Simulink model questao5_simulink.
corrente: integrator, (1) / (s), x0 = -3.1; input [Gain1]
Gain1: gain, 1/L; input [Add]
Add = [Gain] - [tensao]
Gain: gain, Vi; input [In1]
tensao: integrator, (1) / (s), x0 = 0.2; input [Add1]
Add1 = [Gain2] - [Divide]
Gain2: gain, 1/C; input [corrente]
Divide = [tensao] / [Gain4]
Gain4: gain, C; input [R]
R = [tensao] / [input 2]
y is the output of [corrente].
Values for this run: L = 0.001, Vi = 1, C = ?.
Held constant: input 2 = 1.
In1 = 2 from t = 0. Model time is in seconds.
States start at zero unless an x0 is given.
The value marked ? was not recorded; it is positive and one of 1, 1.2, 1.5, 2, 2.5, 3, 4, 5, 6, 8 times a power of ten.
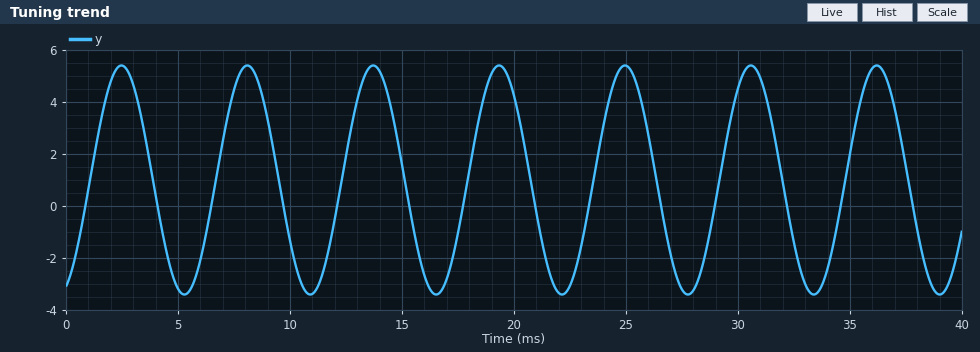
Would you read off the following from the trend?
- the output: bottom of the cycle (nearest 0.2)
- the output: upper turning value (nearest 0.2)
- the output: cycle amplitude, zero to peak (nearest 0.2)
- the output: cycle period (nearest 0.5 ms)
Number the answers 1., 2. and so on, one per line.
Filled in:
1. -3.4
2. 5.4
3. 4.4
4. 5.5 ms
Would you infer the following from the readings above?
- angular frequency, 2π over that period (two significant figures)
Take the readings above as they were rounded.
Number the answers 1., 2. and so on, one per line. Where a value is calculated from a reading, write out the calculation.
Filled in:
1. 2π / 5.5 = 1.1 rad/ms
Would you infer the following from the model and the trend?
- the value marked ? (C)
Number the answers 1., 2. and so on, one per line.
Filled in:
1. 0.0008
